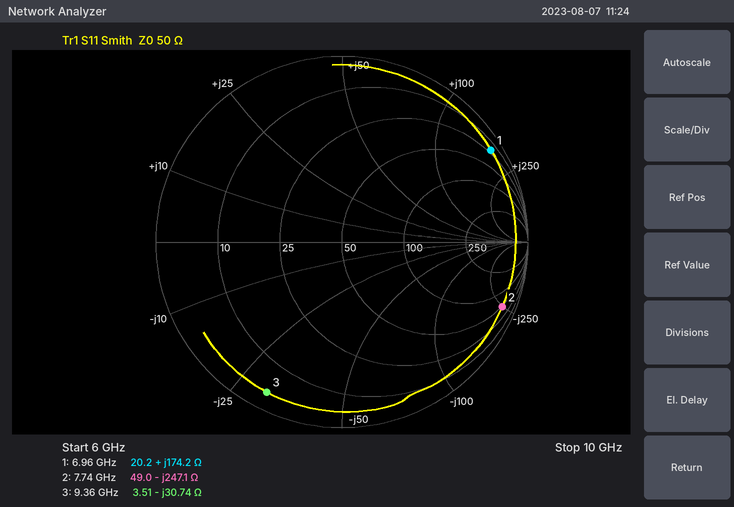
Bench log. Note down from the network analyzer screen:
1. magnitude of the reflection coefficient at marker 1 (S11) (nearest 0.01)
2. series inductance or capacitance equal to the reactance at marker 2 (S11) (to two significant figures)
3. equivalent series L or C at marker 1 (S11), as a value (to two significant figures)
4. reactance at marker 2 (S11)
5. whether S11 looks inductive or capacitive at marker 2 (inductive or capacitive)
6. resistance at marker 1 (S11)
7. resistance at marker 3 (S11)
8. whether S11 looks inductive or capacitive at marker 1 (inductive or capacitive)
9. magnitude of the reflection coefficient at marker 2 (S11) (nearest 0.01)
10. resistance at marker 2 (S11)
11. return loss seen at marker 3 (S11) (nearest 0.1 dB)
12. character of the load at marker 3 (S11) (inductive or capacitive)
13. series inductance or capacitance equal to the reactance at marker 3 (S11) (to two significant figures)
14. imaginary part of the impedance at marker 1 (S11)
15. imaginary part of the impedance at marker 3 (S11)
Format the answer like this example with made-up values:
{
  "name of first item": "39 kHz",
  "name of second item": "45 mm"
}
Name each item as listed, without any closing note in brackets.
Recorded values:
{
  "magnitude of the reflection coefficient at marker 1 (S11)": "0.94",
  "series inductance or capacitance equal to the reactance at marker 2 (S11)": "83 fF",
  "equivalent series L or C at marker 1 (S11), as a value": "4.0 nH",
  "reactance at marker 2": "-247.1 Ω",
  "whether S11 looks inductive or capacitive at marker 2": "capacitive",
  "resistance at marker 1": "20.2 Ω",
  "resistance at marker 3": "3.51 Ω",
  "whether S11 looks inductive or capacitive at marker 1": "inductive",
  "magnitude of the reflection coefficient at marker 2 (S11)": "0.93",
  "resistance at marker 2": "49.0 Ω",
  "return loss seen at marker 3 (S11)": "0.9 dB",
  "character of the load at marker 3 (S11)": "capacitive",
  "series inductance or capacitance equal to the reactance at marker 3 (S11)": "550 fF",
  "imaginary part of the impedance at marker 1": "+174.2 Ω",
  "imaginary part of the impedance at marker 3": "-30.74 Ω"
}
